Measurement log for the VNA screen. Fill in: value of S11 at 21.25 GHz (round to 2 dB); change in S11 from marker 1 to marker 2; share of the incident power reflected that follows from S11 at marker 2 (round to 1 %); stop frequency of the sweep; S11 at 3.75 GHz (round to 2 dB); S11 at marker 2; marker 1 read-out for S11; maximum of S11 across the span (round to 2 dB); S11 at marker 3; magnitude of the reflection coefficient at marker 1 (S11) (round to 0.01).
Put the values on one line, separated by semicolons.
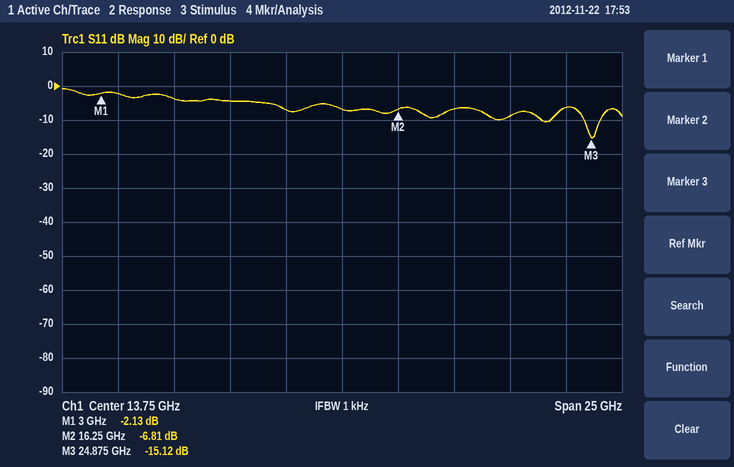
-8 dB; -4.68 dB; 21 %; 26.25 GHz; -2 dB; -6.81 dB; -2.13 dB; 0 dB; -15.12 dB; 0.78
